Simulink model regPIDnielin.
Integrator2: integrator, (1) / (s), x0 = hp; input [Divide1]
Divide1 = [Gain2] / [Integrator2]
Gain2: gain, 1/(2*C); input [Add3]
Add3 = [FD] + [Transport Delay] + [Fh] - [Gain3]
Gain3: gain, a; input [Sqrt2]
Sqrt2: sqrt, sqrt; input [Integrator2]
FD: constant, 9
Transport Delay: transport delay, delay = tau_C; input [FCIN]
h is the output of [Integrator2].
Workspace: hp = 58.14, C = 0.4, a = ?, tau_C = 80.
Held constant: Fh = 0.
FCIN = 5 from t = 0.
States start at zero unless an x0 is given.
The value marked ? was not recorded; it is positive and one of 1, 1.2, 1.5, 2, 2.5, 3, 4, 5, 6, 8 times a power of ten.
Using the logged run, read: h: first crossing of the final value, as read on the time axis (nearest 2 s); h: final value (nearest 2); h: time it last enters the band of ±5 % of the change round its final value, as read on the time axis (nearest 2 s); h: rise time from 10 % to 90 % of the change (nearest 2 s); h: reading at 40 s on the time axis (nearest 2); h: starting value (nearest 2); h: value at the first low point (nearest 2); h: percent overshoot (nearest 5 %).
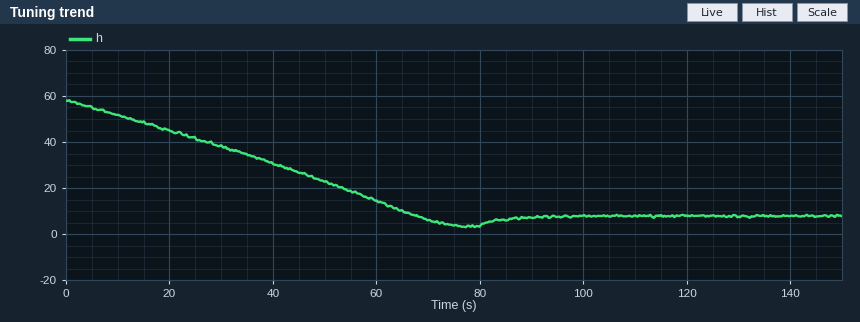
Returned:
68 s
8
82 s
54 s
30
58
4
10 %
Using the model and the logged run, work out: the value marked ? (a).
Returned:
5
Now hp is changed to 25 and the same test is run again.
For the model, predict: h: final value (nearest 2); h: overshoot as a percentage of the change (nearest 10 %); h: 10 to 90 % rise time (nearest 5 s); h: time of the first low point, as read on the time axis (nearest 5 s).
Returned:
8
30 %
15 s
80 s
